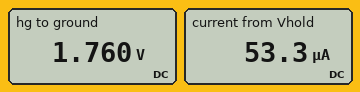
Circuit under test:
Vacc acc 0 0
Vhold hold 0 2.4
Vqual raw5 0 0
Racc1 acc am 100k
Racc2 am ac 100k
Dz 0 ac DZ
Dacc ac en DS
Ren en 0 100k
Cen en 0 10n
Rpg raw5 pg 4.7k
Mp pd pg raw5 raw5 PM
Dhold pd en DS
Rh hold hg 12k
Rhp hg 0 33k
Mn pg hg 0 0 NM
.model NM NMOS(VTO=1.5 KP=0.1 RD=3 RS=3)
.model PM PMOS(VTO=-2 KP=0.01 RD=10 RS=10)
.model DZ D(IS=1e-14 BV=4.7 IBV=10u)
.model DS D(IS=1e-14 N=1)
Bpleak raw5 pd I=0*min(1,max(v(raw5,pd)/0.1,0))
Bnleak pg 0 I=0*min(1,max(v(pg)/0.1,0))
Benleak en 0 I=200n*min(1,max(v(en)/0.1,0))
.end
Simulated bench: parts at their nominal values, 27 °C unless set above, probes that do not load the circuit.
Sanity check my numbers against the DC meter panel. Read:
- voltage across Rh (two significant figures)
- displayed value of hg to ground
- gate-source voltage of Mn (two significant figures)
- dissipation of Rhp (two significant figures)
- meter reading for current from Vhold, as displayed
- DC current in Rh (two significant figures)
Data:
640 mV
1.760 V
1.8 V
94 µW
53.3 µA
53 µA
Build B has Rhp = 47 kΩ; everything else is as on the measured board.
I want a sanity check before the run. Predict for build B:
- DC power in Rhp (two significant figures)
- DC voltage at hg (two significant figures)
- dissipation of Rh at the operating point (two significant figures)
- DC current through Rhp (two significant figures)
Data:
78 µW
1.9 V
20 µW
41 µA
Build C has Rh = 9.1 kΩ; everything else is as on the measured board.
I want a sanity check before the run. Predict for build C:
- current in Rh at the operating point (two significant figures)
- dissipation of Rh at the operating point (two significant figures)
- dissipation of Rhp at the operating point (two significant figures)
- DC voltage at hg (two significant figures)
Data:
57 µA
30 µW
110 µW
1.9 V
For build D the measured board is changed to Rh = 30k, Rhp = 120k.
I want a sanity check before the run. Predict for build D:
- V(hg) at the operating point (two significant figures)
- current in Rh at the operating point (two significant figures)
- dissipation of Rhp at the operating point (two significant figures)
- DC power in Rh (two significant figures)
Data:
1.9 V
16 µA
31 µW
7.7 µW
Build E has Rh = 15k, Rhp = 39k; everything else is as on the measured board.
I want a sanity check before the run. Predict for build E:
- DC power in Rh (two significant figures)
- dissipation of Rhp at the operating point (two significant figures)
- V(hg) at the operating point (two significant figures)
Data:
30 µW
77 µW
1.7 V
